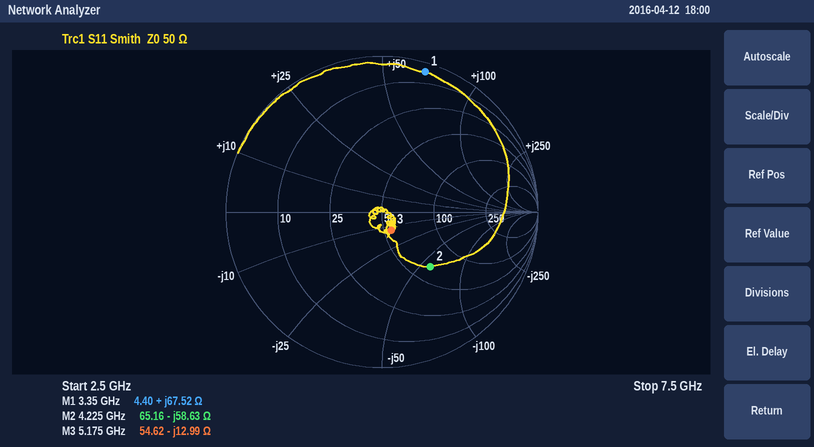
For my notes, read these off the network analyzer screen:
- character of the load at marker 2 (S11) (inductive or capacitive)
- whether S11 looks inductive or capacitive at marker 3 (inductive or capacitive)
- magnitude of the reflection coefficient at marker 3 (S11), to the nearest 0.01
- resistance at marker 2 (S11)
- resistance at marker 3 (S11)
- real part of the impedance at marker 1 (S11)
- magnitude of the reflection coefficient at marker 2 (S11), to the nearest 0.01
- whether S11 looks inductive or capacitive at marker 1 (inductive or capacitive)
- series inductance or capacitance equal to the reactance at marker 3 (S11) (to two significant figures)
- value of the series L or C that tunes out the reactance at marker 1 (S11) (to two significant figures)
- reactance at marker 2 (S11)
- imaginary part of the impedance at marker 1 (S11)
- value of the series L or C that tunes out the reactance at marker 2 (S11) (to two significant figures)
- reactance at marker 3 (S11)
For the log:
capacitive
capacitive
0.13
65.16 Ω
54.62 Ω
4.40 Ω
0.47
inductive
2.4 pF
700 fF
-58.63 Ω
+67.52 Ω
2.2 nH
-12.99 Ω
